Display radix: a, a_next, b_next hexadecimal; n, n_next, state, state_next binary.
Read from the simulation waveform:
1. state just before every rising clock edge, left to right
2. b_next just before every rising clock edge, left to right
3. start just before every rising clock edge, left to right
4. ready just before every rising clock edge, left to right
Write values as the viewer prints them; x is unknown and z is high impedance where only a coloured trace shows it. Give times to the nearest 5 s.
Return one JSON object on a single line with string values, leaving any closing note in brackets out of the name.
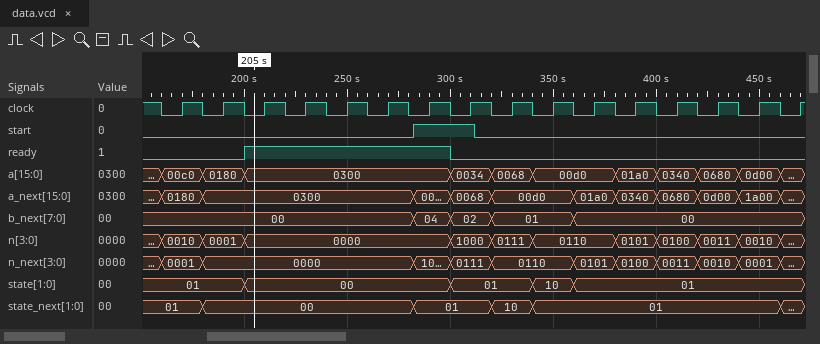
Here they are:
{"state just before every rising clock edge, left to right": "01, 01, 00, 00, 00, 00, 00, 01, 01, 10, 01, 01, 01, 01, 01, 01", "b_next just before every rising clock edge, left to right": "00, 00, 00, 00, 00, 00, 04, 02, 01, 01, 00, 00, 00, 00, 00, 00", "start just before every rising clock edge, left to right": "0 0 0 0 0 0 1 1 0 0 0 0 0 0 0 0", "ready just before every rising clock edge, left to right": "0 0 1 1 1 1 1 0 0 0 0 0 0 0 0 0"}
